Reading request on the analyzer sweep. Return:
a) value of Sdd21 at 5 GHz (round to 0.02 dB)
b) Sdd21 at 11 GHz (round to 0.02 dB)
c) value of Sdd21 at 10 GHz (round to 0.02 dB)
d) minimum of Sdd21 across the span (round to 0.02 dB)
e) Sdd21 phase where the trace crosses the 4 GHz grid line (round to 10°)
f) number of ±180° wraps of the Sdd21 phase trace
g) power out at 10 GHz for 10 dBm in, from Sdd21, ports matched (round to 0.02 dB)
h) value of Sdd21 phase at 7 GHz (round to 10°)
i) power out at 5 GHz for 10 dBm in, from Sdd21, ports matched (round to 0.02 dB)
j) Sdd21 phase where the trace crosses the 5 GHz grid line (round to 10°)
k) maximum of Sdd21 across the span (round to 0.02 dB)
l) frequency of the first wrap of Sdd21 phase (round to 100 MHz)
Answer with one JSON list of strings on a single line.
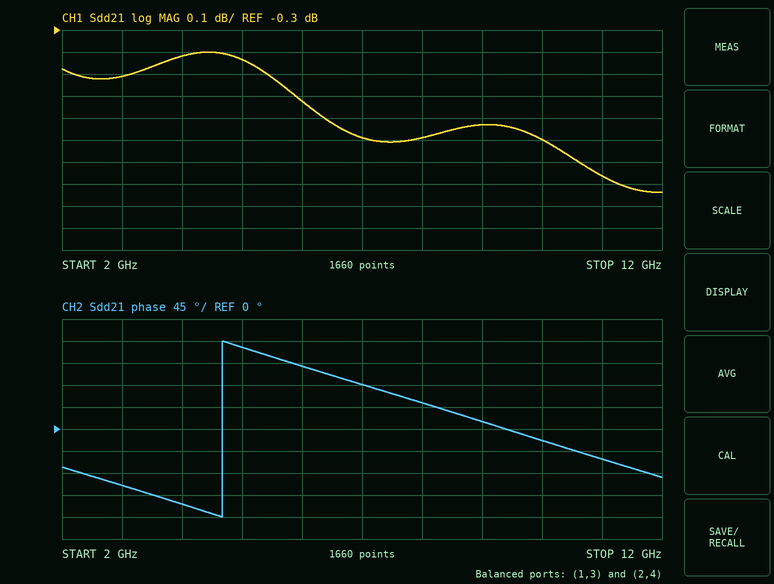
["-0.44 dB", "-0.96 dB", "-0.80 dB", "-1.04 dB", "-150°", "1", "9.20 dBm", "90°", "9.56 dBm", "170°", "-0.40 dB", "4.7 GHz"]
